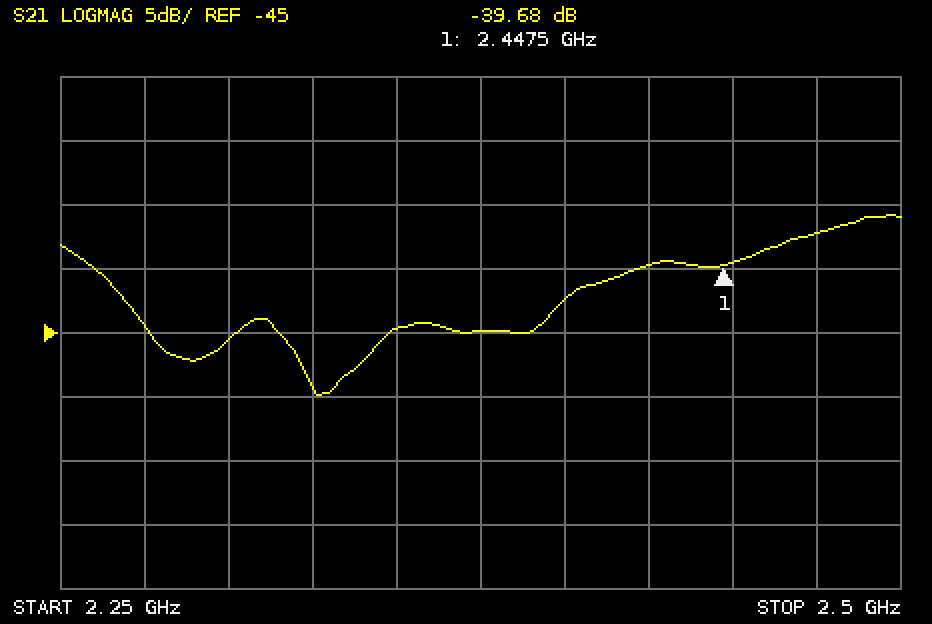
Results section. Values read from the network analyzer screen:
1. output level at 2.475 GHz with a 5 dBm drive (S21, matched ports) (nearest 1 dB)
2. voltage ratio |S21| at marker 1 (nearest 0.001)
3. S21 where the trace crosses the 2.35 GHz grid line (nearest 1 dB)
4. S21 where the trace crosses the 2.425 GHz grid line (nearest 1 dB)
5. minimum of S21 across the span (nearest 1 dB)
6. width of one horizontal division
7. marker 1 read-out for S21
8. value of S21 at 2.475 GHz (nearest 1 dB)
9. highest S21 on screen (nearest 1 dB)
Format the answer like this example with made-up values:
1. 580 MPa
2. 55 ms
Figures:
1. -32 dBm
2. 0.010
3. -45 dB
4. -40 dB
5. -50 dB
6. 25 MHz
7. -39.68 dB
8. -37 dB
9. -36 dB
